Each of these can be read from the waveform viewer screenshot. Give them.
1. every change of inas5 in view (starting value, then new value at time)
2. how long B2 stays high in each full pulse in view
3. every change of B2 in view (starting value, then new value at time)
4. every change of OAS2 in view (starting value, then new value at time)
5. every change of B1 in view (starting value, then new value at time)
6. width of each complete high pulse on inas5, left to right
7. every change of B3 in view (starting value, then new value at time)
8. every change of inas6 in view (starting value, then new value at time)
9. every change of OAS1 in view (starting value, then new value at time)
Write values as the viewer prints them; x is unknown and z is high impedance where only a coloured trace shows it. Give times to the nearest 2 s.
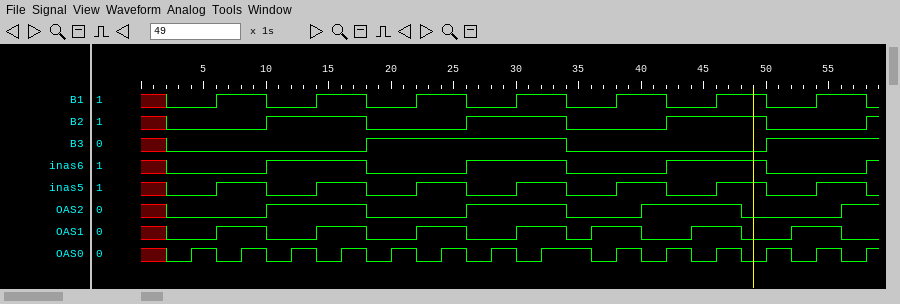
x, 0 at 2 s, 1 at 6 s, 0 at 10 s, 1 at 14 s, 0 at 18 s, 1 at 22 s, 0 at 26 s, 1 at 30 s, 0 at 34 s, 1 at 38 s, 0 at 42 s, 1 at 46 s, 0 at 50 s, 1 at 54 s, 0 at 58 s
8 s, 8 s, 8 s
x, 0 at 2 s, 1 at 10 s, 0 at 18 s, 1 at 26 s, 0 at 34 s, 1 at 42 s, 0 at 50 s, 1 at 58 s
x, 0 at 2 s, 1 at 10 s, 0 at 18 s, 1 at 26 s, 0 at 34 s, 1 at 40 s, 0 at 48 s, 1 at 56 s
x, 0 at 2 s, 1 at 6 s, 0 at 10 s, 1 at 14 s, 0 at 18 s, 1 at 22 s, 0 at 26 s, 1 at 30 s, 0 at 34 s, 1 at 38 s, 0 at 42 s, 1 at 46 s, 0 at 50 s, 1 at 54 s, 0 at 58 s
4 s, 4 s, 4 s, 4 s, 4 s, 4 s, 4 s
x, 0 at 2 s, 1 at 18 s, 0 at 34 s, 1 at 50 s
x, 0 at 2 s, 1 at 10 s, 0 at 18 s, 1 at 26 s, 0 at 34 s, 1 at 42 s, 0 at 50 s, 1 at 58 s
x, 0 at 2 s, 1 at 6 s, 0 at 10 s, 1 at 14 s, 0 at 18 s, 1 at 22 s, 0 at 26 s, 1 at 30 s, 0 at 34 s, 1 at 36 s, 0 at 40 s, 1 at 44 s, 0 at 48 s, 1 at 52 s, 0 at 56 s
